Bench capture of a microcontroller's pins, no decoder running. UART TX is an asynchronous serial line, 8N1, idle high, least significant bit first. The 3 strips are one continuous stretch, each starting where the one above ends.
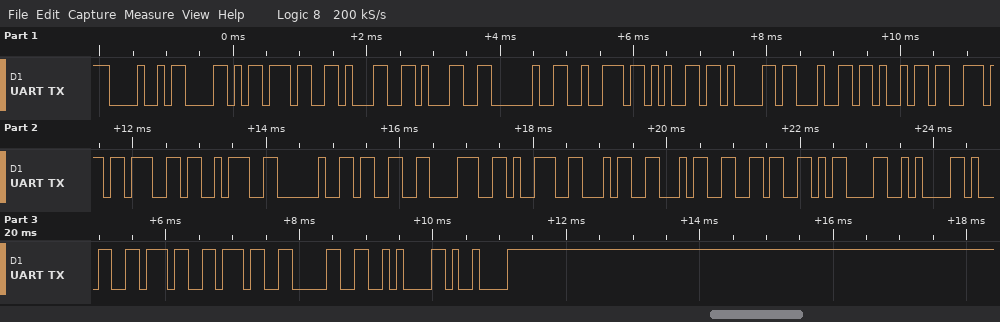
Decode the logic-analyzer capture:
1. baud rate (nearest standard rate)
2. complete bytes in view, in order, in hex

9600 baud
0x48 0x58 0x37 0x31 0x31 0x20 0x72 0x65 0x61 0x64 0x69 0x6E 0x67 0x3A 0x20 0x33 0x38 0x39 0x34 0x34 0x36 0x0D 0x0A 0x31 0x37 0x37 0x30 0x0A 0x09
